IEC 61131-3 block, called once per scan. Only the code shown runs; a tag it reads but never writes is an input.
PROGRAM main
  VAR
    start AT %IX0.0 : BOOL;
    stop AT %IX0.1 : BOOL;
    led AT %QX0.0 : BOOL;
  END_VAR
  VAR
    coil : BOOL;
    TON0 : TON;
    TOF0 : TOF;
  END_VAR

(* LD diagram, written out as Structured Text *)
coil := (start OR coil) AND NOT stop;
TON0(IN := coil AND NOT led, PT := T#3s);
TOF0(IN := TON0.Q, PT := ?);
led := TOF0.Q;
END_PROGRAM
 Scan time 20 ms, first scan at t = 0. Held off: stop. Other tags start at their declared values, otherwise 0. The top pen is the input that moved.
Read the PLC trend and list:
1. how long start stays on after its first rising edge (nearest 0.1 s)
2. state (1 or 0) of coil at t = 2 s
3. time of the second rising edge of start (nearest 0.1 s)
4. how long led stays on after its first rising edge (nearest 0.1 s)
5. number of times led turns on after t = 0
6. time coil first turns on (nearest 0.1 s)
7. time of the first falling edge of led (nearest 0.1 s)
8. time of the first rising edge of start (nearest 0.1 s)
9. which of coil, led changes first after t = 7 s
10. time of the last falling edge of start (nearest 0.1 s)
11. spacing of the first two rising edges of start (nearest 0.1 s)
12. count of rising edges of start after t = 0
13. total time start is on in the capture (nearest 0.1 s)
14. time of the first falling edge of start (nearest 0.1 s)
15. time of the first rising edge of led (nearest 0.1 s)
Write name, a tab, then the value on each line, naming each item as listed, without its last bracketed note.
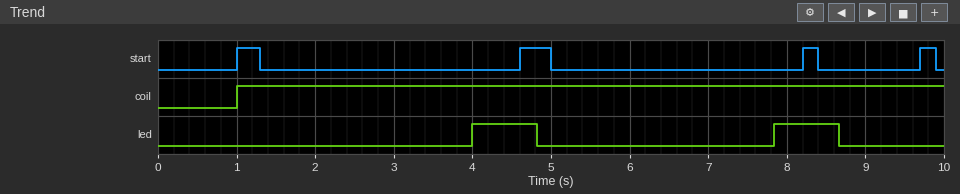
how long start stays on after its first rising edge	0.3 s
state (1 or 0) of coil at t = 2 s	1
time of the second rising edge of start	4.6 s
how long led stays on after its first rising edge	0.8 s
number of times led turns on after t = 0	2
time coil first turns on	1.0 s
time of the first falling edge of led	4.8 s
time of the first rising edge of start	1.0 s
which of coil, led changes first after t = 7 s	led
time of the last falling edge of start	9.9 s
spacing of the first two rising edges of start	3.6 s
count of rising edges of start after t = 0	4
total time start is on in the capture	1.1 s
time of the first falling edge of start	1.3 s
time of the first rising edge of led	4.0 s
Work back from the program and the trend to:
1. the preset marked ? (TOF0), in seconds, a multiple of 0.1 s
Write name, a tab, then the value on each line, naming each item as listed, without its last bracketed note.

the preset marked ? (TOF0), in seconds, a multiple of 0.1 s	0.8 s
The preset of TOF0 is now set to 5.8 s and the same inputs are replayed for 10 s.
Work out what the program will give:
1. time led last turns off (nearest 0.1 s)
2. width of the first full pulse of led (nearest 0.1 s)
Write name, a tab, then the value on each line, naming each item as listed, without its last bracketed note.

time led last turns off	9.8 s
width of the first full pulse of led	5.8 s
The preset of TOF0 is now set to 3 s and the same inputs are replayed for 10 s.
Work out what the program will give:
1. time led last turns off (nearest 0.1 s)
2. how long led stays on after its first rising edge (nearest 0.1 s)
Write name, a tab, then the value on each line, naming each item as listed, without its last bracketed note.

time led last turns off	7.0 s
how long led stays on after its first rising edge	3.0 s
